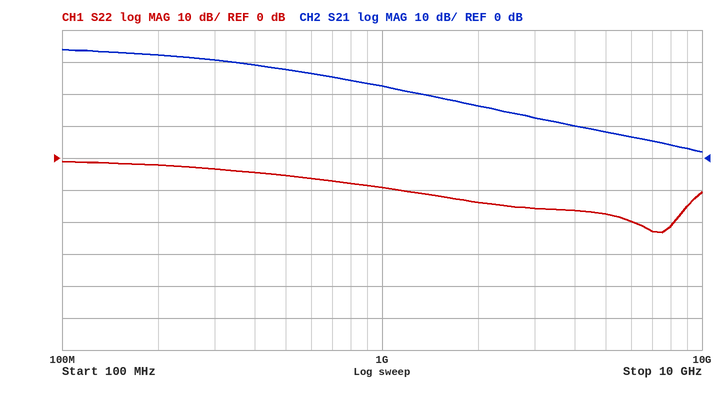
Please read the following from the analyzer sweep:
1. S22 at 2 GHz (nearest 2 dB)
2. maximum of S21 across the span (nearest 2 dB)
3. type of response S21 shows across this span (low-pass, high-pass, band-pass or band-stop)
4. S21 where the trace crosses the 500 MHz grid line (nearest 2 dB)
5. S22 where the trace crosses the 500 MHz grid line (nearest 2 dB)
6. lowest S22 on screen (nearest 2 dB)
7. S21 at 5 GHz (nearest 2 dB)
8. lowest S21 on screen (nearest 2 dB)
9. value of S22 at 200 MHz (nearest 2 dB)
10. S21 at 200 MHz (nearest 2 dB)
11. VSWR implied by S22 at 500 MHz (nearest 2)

-14 dB
34 dB
low-pass
28 dB
-6 dB
-24 dB
8 dB
2 dB
-2 dB
32 dB
4
